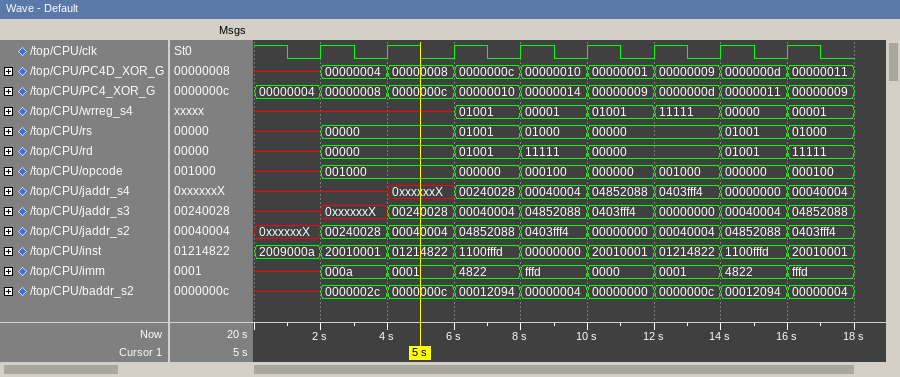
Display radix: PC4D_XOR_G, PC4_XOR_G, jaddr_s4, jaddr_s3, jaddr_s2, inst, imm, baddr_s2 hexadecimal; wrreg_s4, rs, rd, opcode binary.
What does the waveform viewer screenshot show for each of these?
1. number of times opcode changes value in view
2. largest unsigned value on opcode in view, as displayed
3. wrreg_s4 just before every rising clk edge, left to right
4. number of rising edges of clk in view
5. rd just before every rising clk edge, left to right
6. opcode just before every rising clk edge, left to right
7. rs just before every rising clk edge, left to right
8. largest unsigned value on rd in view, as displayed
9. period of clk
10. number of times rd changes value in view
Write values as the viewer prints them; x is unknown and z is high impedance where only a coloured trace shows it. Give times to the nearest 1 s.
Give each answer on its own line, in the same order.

7
001000
x, x, x, 01001, 00001, 01001, 11111, 00000
8
x, 00000, 00000, 01001, 11111, 00000, 00000, 01001
x, 001000, 001000, 000000, 000100, 000000, 001000, 000000
x, 00000, 00000, 01001, 01000, 00000, 00000, 01001
11111
2 s
6
